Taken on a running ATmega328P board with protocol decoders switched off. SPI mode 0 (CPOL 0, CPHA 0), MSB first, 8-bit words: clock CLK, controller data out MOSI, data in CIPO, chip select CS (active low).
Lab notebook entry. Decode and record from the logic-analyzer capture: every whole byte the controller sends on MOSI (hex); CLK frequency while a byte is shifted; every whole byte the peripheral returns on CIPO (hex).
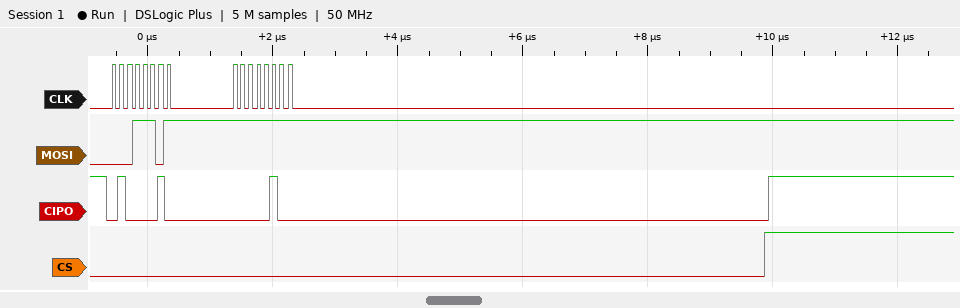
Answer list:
1D FF
8 MHz
42 04
